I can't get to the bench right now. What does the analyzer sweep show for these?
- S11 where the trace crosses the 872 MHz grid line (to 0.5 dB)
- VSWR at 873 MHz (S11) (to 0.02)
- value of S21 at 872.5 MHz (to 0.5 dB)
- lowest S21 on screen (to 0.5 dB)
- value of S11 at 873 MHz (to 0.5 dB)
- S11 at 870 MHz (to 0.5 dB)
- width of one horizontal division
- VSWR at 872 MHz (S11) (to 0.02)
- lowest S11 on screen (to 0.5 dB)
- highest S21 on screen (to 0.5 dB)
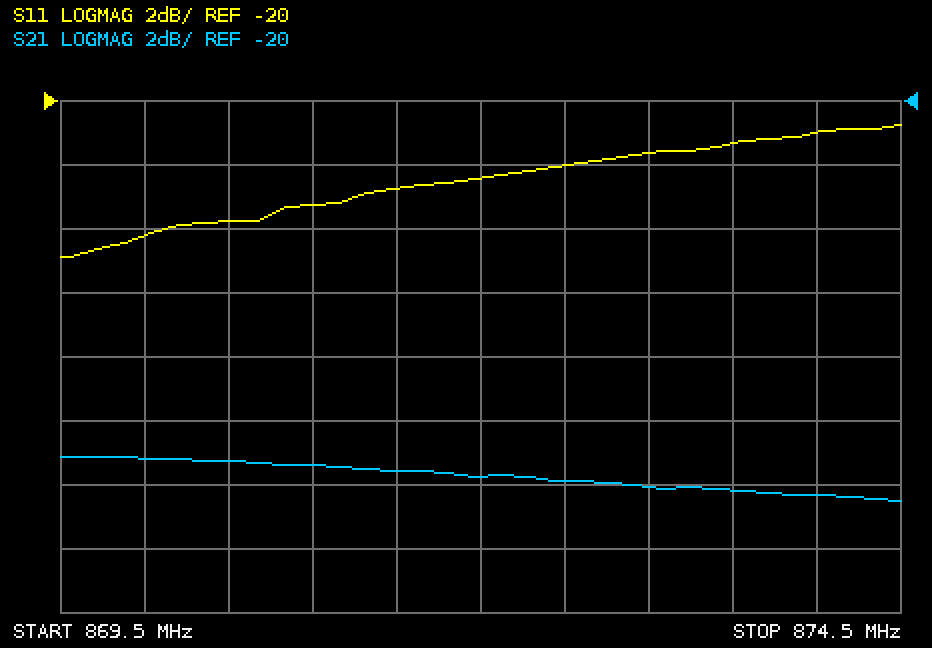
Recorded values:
-22.5 dB
1.18
-32.0 dB
-32.5 dB
-21.5 dB
-24.0 dB
500 kHz
1.16
-25.0 dB
-31.0 dB
